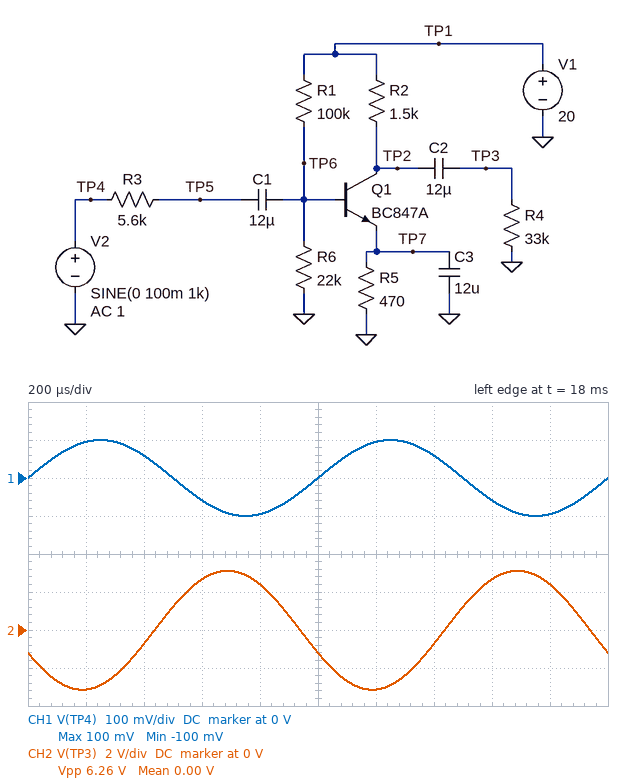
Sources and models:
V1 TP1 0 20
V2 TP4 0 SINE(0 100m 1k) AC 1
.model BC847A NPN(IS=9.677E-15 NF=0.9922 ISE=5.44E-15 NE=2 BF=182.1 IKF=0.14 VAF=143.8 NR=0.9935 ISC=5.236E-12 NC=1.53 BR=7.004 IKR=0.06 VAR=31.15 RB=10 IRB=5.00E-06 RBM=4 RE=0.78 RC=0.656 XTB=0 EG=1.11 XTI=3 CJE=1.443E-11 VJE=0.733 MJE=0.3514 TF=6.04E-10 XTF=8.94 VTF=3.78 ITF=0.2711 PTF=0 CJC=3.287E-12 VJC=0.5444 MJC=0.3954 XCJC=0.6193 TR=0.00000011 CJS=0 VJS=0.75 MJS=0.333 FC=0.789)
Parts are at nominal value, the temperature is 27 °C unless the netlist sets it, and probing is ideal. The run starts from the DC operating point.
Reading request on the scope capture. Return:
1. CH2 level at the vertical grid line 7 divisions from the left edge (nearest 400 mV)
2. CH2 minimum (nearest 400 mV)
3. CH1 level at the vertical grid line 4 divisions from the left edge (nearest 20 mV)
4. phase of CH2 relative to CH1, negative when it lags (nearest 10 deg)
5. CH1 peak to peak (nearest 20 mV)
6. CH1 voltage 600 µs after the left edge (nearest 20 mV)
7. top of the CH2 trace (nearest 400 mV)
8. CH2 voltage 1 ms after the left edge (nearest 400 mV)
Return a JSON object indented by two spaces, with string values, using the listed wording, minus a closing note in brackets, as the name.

{
  "CH2 level at the vertical grid line 7 divisions from the left edge": "-800 mV",
  "CH2 minimum": "-3.2 V",
  "CH1 level at the vertical grid line 4 divisions from the left edge": "-100 mV",
  "phase of CH2 relative to CH1, negative when it lags": "-160 deg",
  "CH1 peak to peak": "200 mV",
  "CH1 voltage 600 µs after the left edge": "-60 mV",
  "top of the CH2 trace": "3.2 V",
  "CH2 voltage 1 ms after the left edge": "-1.2 V"
}
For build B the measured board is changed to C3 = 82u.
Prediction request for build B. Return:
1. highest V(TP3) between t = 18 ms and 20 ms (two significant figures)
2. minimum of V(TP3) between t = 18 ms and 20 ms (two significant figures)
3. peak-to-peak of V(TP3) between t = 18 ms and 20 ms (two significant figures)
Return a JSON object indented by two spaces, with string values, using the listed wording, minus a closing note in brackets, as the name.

{
  "highest V(TP3) between t = 18 ms and 20 ms": "3.4 V",
  "minimum of V(TP3) between t = 18 ms and 20 ms": "-3.4 V",
  "peak-to-peak of V(TP3) between t = 18 ms and 20 ms": "6.8 V"
}
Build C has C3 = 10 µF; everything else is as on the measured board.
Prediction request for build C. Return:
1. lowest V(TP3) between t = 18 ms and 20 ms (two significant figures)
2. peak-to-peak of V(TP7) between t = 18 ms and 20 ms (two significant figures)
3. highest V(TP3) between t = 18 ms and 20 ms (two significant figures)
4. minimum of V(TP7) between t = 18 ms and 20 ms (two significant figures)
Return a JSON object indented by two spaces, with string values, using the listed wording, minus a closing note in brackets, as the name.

{
  "lowest V(TP3) between t = 18 ms and 20 ms": "-3.0 V",
  "peak-to-peak of V(TP7) between t = 18 ms and 20 ms": "68 mV",
  "highest V(TP3) between t = 18 ms and 20 ms": "3.0 V",
  "minimum of V(TP7) between t = 18 ms and 20 ms": "2.4 V"
}
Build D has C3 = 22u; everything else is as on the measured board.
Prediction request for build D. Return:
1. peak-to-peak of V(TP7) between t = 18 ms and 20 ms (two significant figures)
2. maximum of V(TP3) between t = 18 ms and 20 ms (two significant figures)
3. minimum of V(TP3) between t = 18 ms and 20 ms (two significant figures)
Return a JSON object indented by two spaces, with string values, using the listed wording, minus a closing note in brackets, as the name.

{
  "peak-to-peak of V(TP7) between t = 18 ms and 20 ms": "34 mV",
  "maximum of V(TP3) between t = 18 ms and 20 ms": "3.3 V",
  "minimum of V(TP3) between t = 18 ms and 20 ms": "-3.3 V"
}
